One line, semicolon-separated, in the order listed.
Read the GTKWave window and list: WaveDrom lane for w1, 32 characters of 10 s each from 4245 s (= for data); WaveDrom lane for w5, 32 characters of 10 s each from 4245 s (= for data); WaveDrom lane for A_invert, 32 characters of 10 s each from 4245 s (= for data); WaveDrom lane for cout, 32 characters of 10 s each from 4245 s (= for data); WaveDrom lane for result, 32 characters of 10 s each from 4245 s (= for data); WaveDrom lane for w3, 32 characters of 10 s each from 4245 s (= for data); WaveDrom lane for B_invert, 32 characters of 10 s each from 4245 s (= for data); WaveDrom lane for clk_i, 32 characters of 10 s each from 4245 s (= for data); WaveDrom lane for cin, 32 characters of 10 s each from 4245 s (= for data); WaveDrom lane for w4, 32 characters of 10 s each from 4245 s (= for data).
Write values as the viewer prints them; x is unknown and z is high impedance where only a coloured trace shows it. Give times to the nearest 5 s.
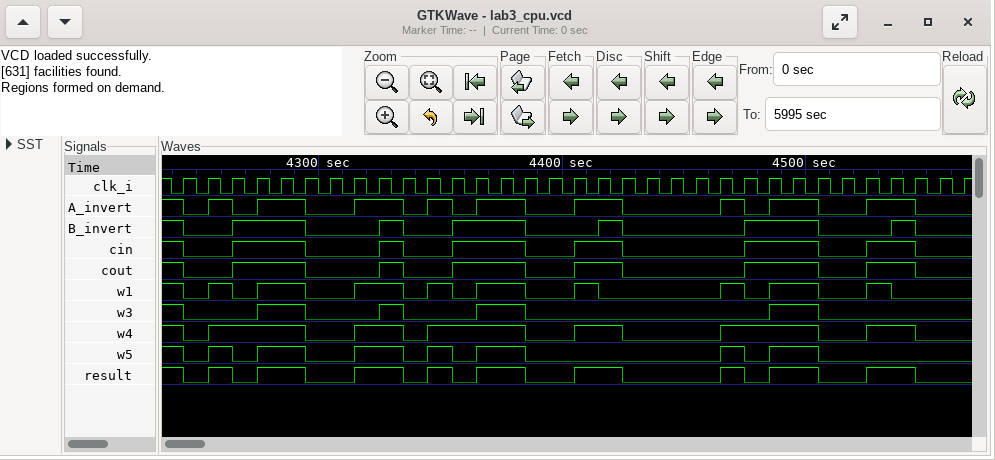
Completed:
{name: 'w1', wave: '0101.0.1.0101.0.10....101.0.10..'}; {name: 'w5', wave: '0101.0.1.0101.0.......101.0.....'}; {name: 'A_invert', wave: '0101.0.1.0101.0.1.0...101.0.1.0.'}; {name: 'cout', wave: '0.1..0..10.1..0.1.0....1..0.1.0.'}; {name: 'result', wave: '0101.0.1.0101.0.1.0...101.0.1.0.'}; {name: 'w3', wave: '0..1.0..10..1.0.........1.0.....'}; {name: 'B_invert', wave: '0.1..0..10.1..0..10....1..0..10.'}; {name: 'clk_i', wave: 'p...............................'}; {name: 'cin', wave: '0.1..0..10.1..0.1.0....1..0.1.0.'}; {name: 'w4', wave: '01...0.1.01...0.1.0...1...0.1.0.'}
